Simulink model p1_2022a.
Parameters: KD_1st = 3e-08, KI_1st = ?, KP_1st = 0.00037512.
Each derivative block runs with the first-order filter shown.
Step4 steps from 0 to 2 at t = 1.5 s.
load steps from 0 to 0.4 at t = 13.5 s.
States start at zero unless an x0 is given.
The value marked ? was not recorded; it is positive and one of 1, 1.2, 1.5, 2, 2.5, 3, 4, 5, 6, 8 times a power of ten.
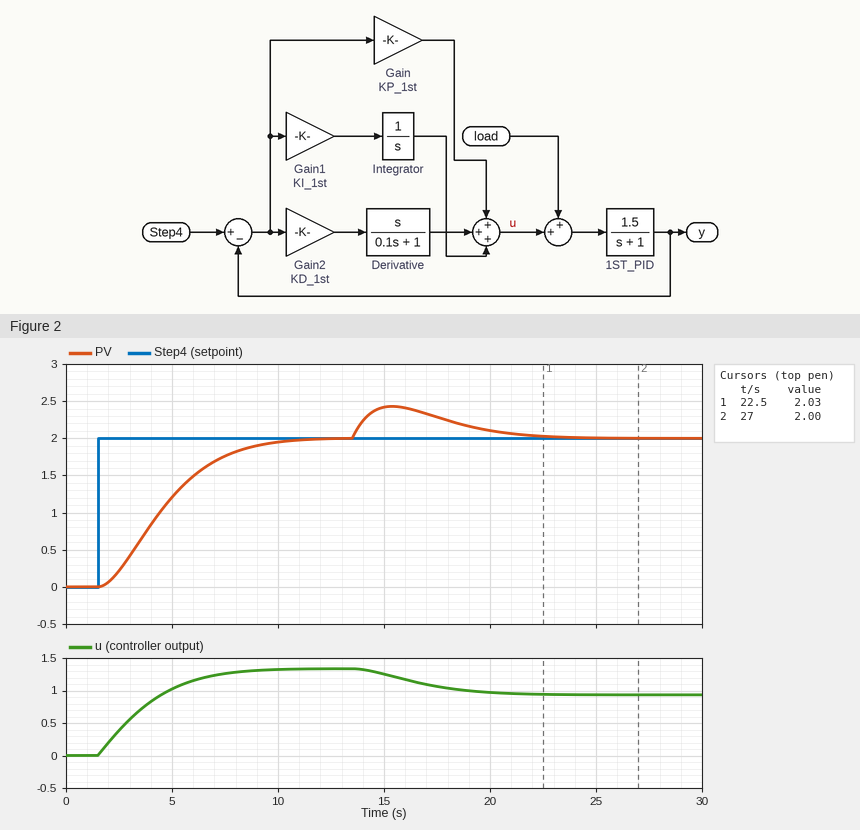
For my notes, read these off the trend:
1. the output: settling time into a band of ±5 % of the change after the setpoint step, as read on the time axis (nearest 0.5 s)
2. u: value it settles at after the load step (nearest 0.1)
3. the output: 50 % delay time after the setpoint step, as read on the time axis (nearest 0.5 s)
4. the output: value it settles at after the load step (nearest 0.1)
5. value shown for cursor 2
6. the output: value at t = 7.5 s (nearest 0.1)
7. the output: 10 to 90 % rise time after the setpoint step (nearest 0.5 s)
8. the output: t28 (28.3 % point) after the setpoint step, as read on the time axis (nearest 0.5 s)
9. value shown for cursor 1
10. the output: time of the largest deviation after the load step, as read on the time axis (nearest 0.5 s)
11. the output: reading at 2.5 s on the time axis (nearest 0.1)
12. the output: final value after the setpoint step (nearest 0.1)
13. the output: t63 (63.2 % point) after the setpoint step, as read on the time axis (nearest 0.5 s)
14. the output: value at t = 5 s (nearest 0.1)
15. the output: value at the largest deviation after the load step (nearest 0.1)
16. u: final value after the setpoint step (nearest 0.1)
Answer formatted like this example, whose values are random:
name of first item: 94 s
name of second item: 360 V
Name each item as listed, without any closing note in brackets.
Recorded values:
the output: settling time into a band of ±5 % of the change after the setpoint step, as read on the time axis: 9.0 s
u: value it settles at after the load step: 0.9
the output: 50 % delay time after the setpoint step, as read on the time axis: 4.5 s
the output: value it settles at after the load step: 2.0
value shown for cursor 2: 2.00
the output: value at t = 7.5 s: 1.8
the output: 10 to 90 % rise time after the setpoint step: 5.5 s
the output: t28 (28.3 % point) after the setpoint step, as read on the time axis: 3.5 s
value shown for cursor 1: 2.03
the output: time of the largest deviation after the load step, as read on the time axis: 15.5 s
the output: reading at 2.5 s on the time axis: 0.2
the output: final value after the setpoint step: 2.0
the output: t63 (63.2 % point) after the setpoint step, as read on the time axis: 5.0 s
the output: value at t = 5 s: 1.2
the output: value at the largest deviation after the load step: 2.4
u: final value after the setpoint step: 1.3
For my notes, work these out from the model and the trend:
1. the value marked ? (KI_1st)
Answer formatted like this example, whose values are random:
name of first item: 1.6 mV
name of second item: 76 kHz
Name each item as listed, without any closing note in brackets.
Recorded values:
the value marked ?: 0.2
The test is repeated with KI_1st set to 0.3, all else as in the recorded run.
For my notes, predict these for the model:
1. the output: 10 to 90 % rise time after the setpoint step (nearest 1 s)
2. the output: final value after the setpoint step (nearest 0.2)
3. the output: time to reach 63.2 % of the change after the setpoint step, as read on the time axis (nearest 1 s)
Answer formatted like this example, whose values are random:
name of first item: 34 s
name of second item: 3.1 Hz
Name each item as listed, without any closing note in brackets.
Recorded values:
the output: 10 to 90 % rise time after the setpoint step: 3 s
the output: final value after the setpoint step: 2.0
the output: time to reach 63.2 % of the change after the setpoint step, as read on the time axis: 4 s
